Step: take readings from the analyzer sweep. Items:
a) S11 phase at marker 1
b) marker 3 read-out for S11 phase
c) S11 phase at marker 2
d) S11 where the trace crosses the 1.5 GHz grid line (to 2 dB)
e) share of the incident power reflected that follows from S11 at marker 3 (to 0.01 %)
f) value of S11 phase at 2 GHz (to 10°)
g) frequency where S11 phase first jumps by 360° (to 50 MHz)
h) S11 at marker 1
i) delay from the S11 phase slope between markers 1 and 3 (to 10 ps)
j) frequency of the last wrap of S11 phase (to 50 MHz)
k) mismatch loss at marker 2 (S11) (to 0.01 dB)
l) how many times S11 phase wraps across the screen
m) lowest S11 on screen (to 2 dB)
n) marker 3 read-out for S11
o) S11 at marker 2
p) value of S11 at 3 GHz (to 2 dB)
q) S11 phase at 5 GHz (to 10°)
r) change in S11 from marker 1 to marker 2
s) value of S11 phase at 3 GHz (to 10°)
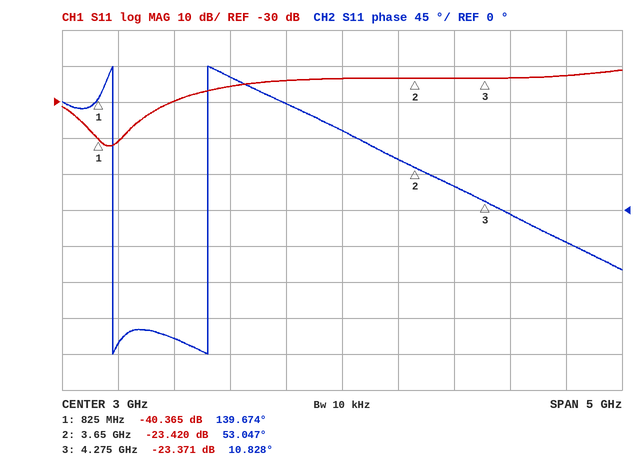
139.674°
10.828°
53.047°
-30 dB
0.46 %
170°
950 MHz
-40.365 dB
100 ps
1.80 GHz
0.02 dB
2
-42 dB
-23.371 dB
-23.420 dB
-24 dB
-40°
16.945 dB
100°
